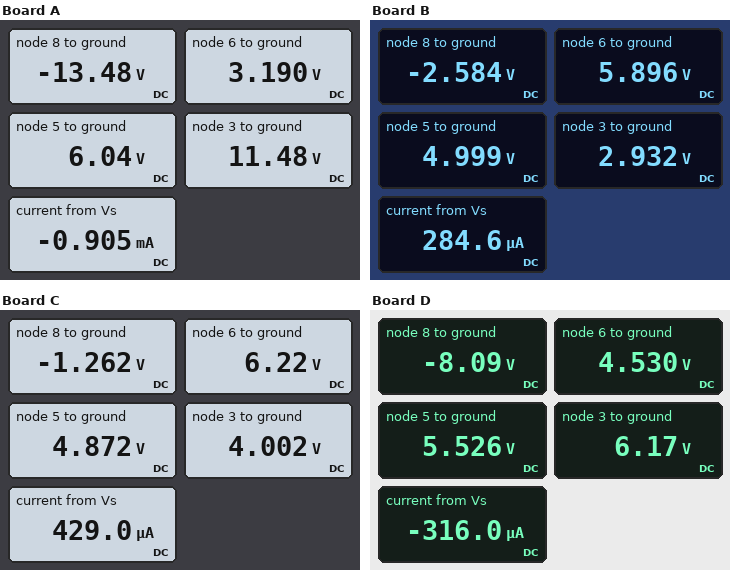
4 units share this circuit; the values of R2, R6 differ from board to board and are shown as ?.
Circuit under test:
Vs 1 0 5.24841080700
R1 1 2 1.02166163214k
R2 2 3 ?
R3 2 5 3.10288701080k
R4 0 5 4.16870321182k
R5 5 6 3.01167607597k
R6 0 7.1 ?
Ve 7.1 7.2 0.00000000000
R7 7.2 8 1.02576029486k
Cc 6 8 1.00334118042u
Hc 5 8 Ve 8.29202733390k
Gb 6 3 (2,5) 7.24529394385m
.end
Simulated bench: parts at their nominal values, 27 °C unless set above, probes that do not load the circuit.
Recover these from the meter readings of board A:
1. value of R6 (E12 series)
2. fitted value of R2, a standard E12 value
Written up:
4.7 kΩ
5.6 kΩ
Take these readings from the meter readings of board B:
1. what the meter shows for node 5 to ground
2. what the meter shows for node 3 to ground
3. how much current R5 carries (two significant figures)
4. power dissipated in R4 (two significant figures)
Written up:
4.999 V
2.932 V
300 µA
6.0 mW
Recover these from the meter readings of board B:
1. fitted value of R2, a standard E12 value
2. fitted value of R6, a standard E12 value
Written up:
6.8 kΩ
1.8 kΩ
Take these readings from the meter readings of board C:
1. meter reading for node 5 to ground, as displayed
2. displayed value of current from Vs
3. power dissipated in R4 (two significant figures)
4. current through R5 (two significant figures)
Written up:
4.872 V
429.0 µA
5.7 mW
450 µA
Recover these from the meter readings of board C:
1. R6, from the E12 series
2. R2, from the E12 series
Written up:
680 Ω
1.8 kΩ
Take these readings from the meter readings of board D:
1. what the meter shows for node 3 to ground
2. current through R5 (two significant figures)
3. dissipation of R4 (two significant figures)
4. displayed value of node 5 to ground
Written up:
6.17 V
330 µA
7.3 mW
5.526 V
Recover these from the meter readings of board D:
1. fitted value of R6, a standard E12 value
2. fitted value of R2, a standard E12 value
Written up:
3.9 kΩ
1.8 kΩ
